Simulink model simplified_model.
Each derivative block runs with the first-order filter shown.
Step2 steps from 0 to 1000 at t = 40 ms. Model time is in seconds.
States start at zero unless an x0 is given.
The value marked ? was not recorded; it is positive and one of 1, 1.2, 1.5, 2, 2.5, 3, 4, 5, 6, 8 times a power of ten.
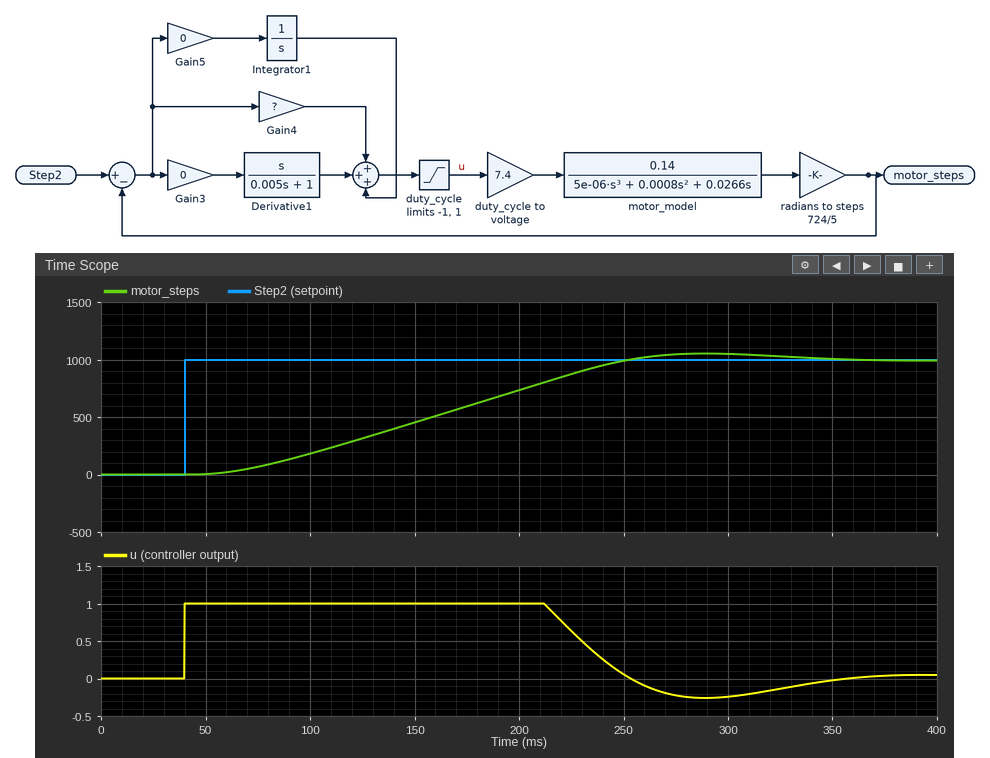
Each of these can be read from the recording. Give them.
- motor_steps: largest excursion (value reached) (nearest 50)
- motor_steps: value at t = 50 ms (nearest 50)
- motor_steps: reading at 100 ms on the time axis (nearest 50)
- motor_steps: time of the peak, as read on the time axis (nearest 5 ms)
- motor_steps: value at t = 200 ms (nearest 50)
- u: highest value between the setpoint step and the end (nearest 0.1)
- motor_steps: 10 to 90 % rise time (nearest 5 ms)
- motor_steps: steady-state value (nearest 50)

1050
0
200
290 ms
750
1.0
145 ms
1000
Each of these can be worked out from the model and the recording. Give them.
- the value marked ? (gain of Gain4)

0.005
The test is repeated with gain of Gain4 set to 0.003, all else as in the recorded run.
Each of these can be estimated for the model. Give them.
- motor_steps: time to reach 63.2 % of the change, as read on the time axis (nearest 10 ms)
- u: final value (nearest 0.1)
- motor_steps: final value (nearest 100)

180 ms
0.0
1000
